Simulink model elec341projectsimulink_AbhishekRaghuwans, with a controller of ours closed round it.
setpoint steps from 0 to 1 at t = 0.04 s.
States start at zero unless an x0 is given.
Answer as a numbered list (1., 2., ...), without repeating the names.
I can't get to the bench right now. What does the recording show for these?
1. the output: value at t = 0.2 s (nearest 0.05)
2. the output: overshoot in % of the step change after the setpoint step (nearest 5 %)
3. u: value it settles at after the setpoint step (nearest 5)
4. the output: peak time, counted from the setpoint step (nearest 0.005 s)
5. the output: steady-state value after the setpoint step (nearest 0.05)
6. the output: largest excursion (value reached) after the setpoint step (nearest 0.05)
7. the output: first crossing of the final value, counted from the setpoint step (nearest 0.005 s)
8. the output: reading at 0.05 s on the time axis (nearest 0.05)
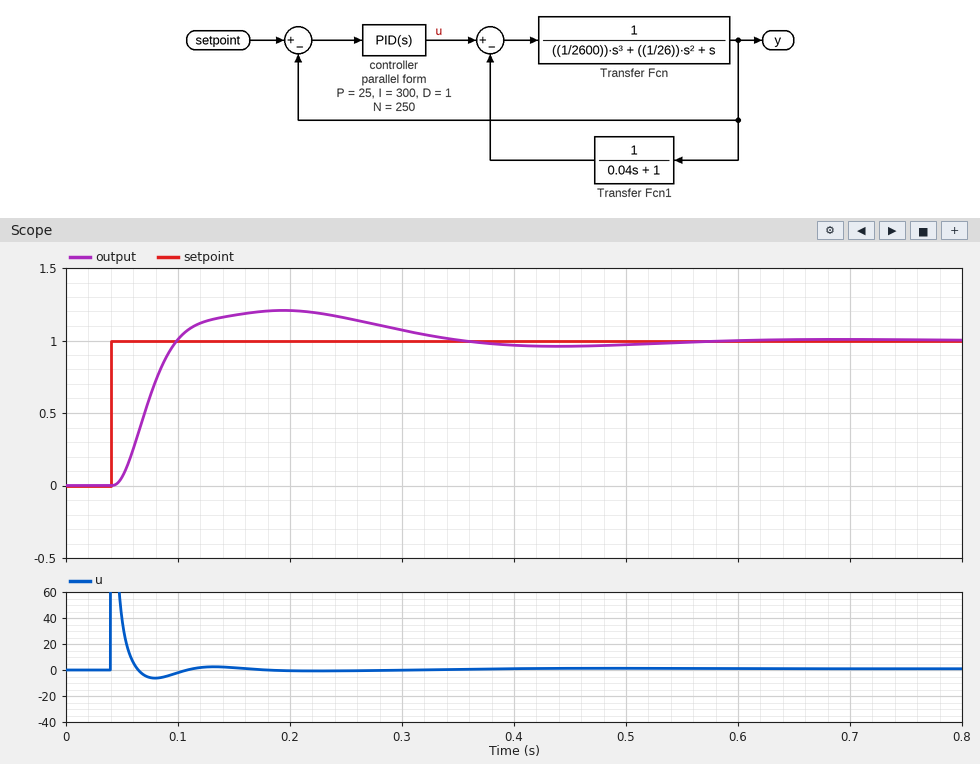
1. 1.20
2. 20 %
3. 0
4. 0.155 s
5. 1.00
6. 1.20
7. 0.060 s
8. 0.05
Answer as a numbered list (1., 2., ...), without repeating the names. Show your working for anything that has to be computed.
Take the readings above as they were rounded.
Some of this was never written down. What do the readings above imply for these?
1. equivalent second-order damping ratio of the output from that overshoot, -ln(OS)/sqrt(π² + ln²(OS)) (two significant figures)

1. ln(0.2) = -1.609; 1.609 / sqrt(9.870 + 2.590) = 0.46
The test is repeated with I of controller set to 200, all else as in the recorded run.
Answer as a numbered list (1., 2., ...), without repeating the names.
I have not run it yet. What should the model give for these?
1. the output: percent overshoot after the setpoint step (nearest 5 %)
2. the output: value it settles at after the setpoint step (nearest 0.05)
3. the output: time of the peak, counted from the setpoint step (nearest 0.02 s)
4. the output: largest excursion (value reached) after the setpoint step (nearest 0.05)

1. 15 %
2. 1.00
3. 0.18 s
4. 1.15
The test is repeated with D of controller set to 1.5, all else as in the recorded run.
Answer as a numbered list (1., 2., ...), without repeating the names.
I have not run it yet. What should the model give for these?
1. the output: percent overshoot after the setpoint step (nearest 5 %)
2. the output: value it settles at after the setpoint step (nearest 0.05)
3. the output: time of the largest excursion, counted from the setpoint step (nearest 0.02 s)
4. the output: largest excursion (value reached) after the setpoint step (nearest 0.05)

1. 15 %
2. 1.00
3. 0.18 s
4. 1.15
